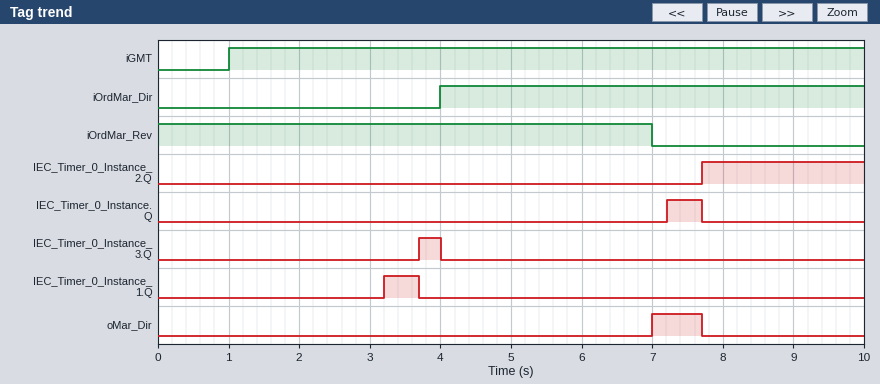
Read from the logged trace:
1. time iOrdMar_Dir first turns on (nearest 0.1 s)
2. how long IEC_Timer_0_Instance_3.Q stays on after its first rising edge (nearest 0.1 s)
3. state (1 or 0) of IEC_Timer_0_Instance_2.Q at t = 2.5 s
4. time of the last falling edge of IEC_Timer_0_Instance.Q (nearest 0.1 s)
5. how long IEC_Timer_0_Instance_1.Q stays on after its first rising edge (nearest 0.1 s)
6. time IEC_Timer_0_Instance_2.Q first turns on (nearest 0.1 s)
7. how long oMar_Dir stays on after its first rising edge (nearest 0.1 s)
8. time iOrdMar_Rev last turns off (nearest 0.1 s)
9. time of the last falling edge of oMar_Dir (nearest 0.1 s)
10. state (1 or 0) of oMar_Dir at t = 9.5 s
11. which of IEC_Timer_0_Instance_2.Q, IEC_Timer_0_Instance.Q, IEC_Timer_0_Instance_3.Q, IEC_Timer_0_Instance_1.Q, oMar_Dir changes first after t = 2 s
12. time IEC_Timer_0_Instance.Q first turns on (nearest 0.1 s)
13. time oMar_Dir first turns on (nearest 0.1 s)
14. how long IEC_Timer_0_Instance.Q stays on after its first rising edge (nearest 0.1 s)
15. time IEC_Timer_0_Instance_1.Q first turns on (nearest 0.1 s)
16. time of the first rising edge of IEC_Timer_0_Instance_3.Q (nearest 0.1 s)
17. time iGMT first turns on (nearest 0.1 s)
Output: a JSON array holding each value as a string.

["4.0 s", "0.3 s", "0", "7.7 s", "0.5 s", "7.7 s", "0.7 s", "7.0 s", "7.7 s", "0", "IEC_Timer_0_Instance_1.Q", "7.2 s", "7.0 s", "0.5 s", "3.2 s", "3.7 s", "1.0 s"]
